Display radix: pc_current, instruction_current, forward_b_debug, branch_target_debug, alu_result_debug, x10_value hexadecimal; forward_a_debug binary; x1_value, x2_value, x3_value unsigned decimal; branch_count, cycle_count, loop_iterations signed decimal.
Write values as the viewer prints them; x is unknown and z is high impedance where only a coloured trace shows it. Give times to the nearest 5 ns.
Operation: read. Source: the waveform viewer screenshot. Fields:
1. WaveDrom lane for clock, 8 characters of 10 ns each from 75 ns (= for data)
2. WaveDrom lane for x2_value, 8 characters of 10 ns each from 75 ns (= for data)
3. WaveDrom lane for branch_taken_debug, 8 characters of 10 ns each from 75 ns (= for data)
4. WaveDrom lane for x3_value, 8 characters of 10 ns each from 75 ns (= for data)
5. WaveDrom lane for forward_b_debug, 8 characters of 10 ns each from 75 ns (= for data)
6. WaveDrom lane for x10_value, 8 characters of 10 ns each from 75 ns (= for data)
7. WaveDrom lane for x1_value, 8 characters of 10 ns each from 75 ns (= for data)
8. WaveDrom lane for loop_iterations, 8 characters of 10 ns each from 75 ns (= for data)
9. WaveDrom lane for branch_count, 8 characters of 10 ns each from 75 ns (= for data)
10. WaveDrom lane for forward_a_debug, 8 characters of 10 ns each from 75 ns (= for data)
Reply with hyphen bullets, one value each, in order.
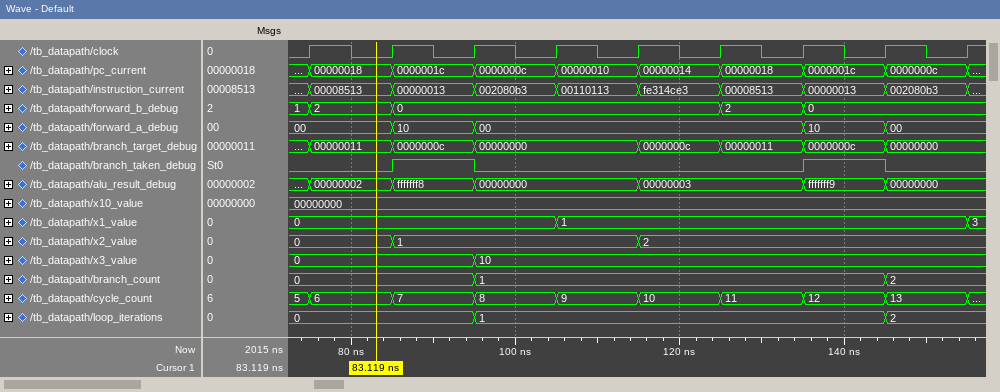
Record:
- {name: 'clock', wave: 'p.......'}
- {name: 'x2_value', wave: '==..=...', data: '0 1 2'}
- {name: 'branch_taken_debug', wave: '010...10'}
- {name: 'x3_value', wave: '=.=.....', data: '0 10'}
- {name: 'forward_b_debug', wave: '==...==.', data: '2 0 2 0'}
- {name: 'x10_value', wave: '=.......', data: '00000000'}
- {name: 'x1_value', wave: '=..=....', data: '0 1'}
- {name: 'loop_iterations', wave: '=.=....=', data: '0 1 2'}
- {name: 'branch_count', wave: '=.=....=', data: '0 1 2'}
- {name: 'forward_a_debug', wave: '===...==', data: '00 10 00 10 00'}
